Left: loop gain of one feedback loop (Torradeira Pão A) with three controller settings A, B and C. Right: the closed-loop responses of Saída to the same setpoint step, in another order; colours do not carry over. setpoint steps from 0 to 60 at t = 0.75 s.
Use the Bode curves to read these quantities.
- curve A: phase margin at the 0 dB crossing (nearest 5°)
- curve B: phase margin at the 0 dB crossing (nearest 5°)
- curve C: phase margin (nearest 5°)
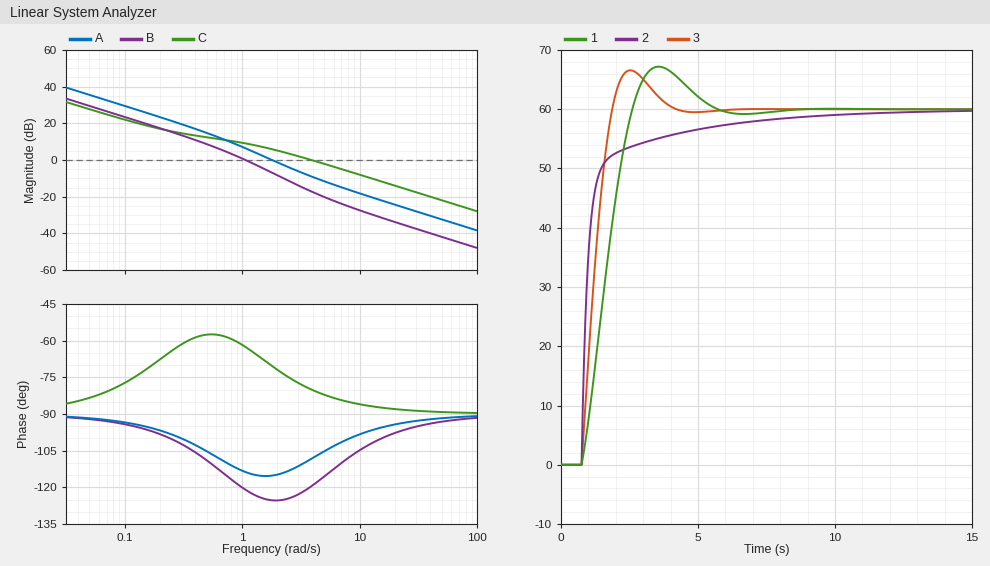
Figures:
65°
60°
100°
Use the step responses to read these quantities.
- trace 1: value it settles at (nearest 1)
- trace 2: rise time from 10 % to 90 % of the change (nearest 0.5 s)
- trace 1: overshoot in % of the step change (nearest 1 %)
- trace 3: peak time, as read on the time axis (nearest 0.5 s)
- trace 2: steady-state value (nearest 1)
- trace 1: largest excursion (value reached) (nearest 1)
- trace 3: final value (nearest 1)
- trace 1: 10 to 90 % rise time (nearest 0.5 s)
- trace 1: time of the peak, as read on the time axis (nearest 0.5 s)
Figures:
60
2.0 s
12 %
2.5 s
60
67
60
1.5 s
3.5 s
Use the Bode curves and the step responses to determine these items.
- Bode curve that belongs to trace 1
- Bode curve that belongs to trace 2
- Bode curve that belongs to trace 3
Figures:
B
C
A
